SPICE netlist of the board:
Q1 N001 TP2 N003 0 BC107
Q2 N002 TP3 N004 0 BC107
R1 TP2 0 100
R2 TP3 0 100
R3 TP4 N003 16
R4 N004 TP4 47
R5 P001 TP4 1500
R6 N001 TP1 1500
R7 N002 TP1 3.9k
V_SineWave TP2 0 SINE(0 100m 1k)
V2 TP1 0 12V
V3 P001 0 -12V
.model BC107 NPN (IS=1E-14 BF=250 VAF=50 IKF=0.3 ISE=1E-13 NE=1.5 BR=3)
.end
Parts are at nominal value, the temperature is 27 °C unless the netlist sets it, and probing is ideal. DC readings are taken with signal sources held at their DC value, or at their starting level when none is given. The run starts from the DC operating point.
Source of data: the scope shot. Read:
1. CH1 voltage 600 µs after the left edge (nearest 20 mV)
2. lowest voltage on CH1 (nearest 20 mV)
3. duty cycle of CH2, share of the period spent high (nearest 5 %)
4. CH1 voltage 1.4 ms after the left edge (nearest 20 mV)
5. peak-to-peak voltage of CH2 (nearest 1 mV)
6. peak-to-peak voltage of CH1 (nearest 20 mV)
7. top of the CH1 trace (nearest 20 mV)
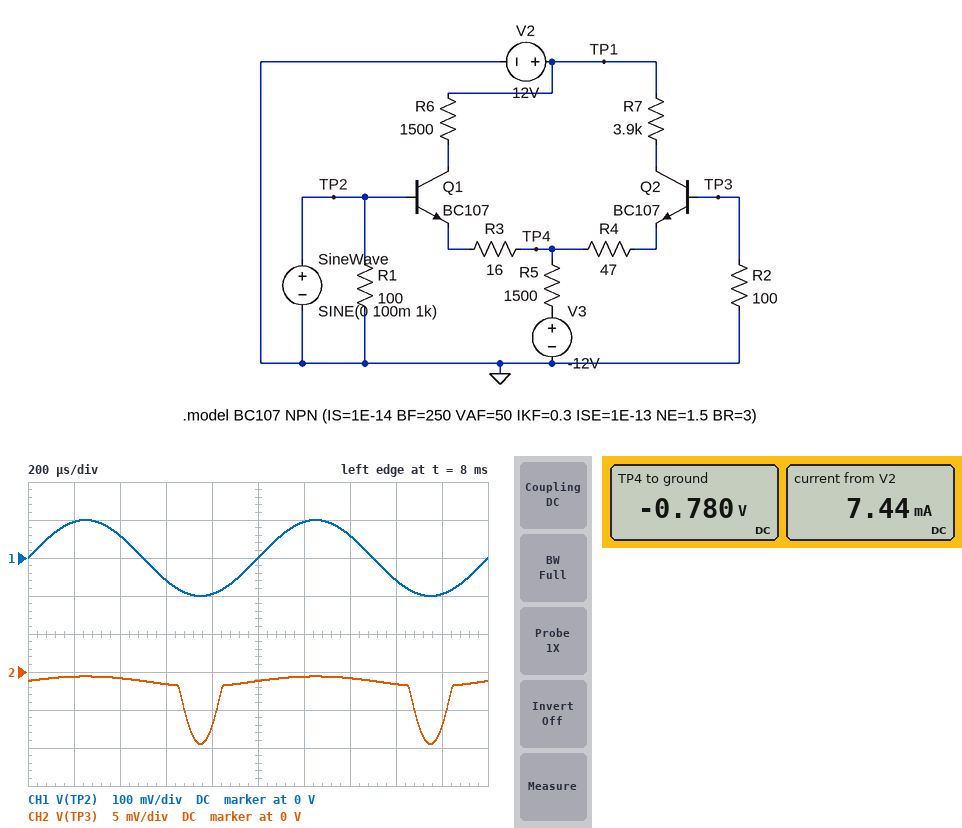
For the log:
-60 mV
-100 mV
85 %
60 mV
9 mV
200 mV
100 mV
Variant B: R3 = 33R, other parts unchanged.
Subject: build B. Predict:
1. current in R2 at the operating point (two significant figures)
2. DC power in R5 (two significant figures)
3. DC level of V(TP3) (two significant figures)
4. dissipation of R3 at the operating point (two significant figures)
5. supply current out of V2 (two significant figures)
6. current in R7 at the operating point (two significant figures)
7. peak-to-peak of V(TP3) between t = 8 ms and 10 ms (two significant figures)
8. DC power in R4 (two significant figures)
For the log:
17 µA
83 mW
-1.7 mV
620 µW
7.4 mA
3.1 mA
40 mV
460 µW
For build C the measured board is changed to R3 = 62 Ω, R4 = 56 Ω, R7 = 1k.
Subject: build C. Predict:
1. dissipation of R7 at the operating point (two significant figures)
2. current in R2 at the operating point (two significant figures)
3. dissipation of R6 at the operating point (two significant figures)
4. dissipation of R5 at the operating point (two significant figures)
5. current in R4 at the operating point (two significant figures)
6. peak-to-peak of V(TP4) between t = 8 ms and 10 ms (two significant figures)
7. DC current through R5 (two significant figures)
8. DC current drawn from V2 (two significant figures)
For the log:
15 mW
18 µA
19 mW
82 mW
3.9 mA
93 mV
7.4 mA
7.4 mA
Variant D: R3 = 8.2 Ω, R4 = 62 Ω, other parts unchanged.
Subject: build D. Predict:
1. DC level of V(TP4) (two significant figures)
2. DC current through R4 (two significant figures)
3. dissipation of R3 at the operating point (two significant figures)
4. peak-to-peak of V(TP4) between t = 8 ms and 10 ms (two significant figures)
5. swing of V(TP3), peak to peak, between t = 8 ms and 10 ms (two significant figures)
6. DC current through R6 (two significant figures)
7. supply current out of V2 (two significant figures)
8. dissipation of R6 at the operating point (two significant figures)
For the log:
-750 mV
1.4 mA
300 µW
170 mV
1.1 mV
6.0 mA
7.5 mA
55 mW
